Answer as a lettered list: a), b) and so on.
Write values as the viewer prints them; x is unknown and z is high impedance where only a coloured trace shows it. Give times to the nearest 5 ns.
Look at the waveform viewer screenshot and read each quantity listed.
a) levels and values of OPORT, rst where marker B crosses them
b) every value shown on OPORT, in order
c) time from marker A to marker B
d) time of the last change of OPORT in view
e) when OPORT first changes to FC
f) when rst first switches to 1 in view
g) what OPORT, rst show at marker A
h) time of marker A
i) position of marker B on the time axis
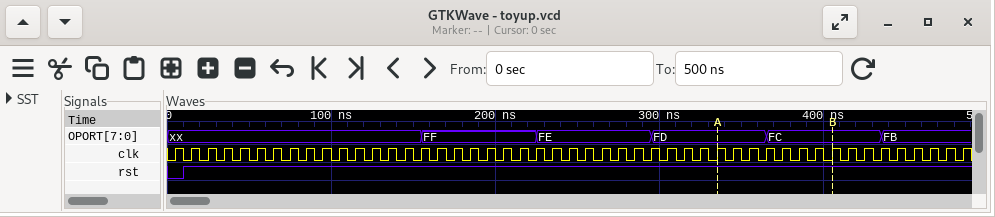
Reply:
a) OPORT=FC, rst=1
b) xx, FF, FE, FD, FC, FB
c) 70 ns
d) 435 ns
e) 365 ns
f) 10 ns
g) OPORT=FD, rst=1
h) 335 ns
i) 405 ns
